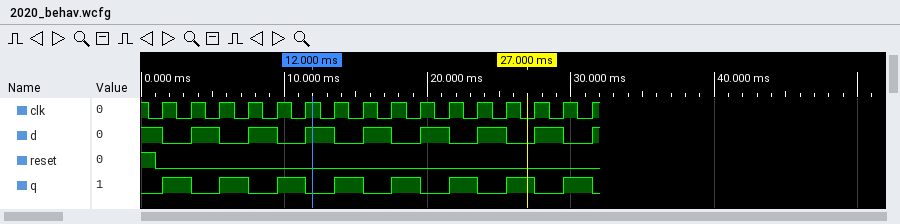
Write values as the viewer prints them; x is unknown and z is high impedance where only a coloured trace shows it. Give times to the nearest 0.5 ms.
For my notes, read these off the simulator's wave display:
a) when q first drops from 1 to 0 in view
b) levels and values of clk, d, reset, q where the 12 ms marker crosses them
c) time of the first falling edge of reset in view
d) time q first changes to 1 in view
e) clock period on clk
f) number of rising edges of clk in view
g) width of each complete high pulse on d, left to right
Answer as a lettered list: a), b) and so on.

a) 3.5 ms
b) clk=1, d=1, reset=0, q=0
c) 1 ms
d) 1.5 ms
e) 2 ms
f) 16
g) 2 ms, 2 ms, 2 ms, 2 ms, 2 ms, 2 ms, 2 ms
